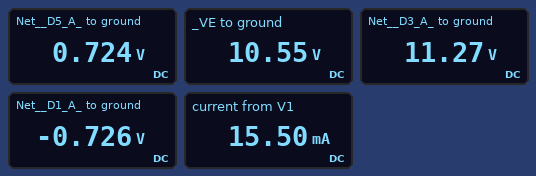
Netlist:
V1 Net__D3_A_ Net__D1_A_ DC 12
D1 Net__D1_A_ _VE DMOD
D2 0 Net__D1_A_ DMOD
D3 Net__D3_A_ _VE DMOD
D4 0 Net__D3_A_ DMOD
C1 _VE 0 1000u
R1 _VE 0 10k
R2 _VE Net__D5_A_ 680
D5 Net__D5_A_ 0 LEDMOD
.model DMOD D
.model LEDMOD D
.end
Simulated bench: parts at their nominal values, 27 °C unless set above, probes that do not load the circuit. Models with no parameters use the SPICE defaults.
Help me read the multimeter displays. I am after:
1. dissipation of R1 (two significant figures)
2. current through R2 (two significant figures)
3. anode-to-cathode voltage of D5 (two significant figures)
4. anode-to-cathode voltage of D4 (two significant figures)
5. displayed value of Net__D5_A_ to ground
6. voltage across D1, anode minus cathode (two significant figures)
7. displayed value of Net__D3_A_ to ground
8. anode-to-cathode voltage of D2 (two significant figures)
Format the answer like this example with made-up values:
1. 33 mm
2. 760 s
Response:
1. 11 mW
2. 14 mA
3. 720 mV
4. -11 V
5. 0.724 V
6. -11 V
7. 11.27 V
8. 730 mV
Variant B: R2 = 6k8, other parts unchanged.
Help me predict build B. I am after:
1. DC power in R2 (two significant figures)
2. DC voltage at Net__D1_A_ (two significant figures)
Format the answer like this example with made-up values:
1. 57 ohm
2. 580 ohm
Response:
1. 15 mW
2. -680 mV
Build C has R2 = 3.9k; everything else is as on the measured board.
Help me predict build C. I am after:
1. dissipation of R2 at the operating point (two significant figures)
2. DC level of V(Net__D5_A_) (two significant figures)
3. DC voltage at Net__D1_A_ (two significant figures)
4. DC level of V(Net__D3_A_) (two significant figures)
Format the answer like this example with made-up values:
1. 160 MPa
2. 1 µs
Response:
1. 25 mW
2. 680 mV
3. -690 mV
4. 11 V
